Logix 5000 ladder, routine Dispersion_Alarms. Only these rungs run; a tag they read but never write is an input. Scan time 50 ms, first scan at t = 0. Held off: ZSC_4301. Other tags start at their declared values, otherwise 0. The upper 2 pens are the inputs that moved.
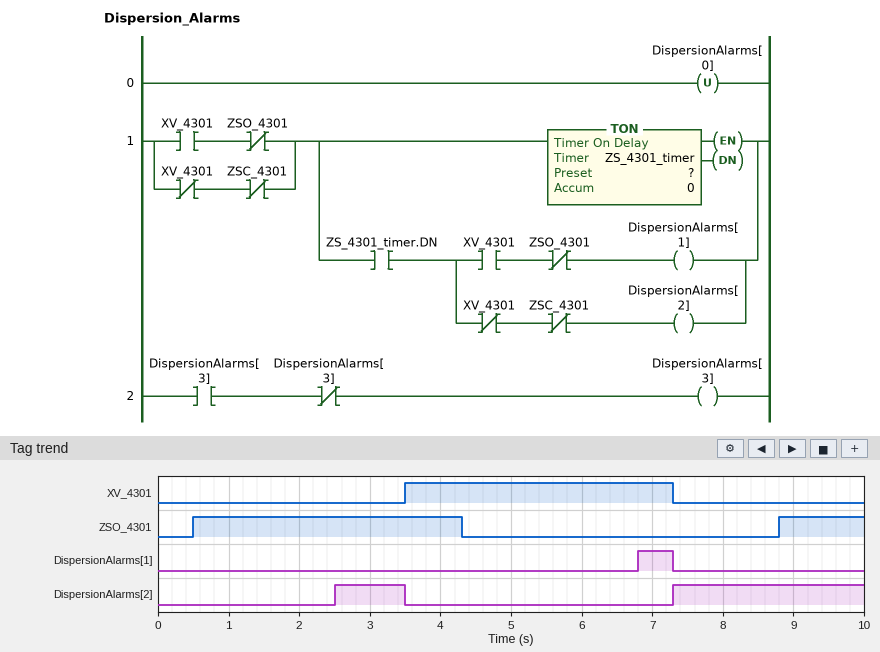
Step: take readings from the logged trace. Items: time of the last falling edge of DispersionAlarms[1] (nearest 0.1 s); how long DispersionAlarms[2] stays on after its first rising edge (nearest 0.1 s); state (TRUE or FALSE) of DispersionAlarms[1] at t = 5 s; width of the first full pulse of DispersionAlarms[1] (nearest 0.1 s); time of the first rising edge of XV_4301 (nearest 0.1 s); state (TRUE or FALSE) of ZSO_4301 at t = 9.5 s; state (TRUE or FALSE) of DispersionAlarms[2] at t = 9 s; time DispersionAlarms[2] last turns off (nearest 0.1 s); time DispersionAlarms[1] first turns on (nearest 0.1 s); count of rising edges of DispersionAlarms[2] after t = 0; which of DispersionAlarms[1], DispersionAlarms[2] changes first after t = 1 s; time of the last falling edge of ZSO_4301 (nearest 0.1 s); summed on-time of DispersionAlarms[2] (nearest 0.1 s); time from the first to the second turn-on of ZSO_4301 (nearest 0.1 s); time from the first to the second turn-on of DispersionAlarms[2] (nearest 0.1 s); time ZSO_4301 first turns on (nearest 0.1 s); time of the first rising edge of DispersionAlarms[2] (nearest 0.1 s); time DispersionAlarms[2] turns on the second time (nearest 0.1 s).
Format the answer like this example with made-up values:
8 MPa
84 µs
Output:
7.3 s
1.0 s
FALSE
0.5 s
3.5 s
TRUE
TRUE
3.5 s
6.8 s
2
DispersionAlarms[2]
4.3 s
3.7 s
8.3 s
4.8 s
0.5 s
2.5 s
7.3 s
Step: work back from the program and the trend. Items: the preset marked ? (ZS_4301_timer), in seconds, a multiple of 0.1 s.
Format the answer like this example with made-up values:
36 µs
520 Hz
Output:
2.5 s
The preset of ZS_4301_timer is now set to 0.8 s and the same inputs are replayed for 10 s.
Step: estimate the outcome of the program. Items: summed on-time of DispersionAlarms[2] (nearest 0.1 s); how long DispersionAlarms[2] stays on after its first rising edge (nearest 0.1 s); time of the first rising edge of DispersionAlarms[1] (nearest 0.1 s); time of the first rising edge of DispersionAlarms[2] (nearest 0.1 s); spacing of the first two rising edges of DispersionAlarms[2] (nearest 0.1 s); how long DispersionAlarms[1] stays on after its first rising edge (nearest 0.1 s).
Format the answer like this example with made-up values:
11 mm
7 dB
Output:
5.4 s
2.7 s
5.1 s
0.8 s
6.5 s
2.2 s
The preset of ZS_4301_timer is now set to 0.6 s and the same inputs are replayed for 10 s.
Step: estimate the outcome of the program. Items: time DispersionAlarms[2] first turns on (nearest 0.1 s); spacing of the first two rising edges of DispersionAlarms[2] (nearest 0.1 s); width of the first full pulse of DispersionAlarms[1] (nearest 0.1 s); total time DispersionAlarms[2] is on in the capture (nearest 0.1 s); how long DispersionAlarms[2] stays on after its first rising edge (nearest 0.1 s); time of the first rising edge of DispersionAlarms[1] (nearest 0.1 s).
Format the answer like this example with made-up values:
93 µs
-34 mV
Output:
0.6 s
6.7 s
2.4 s
5.6 s
2.9 s
4.9 s
